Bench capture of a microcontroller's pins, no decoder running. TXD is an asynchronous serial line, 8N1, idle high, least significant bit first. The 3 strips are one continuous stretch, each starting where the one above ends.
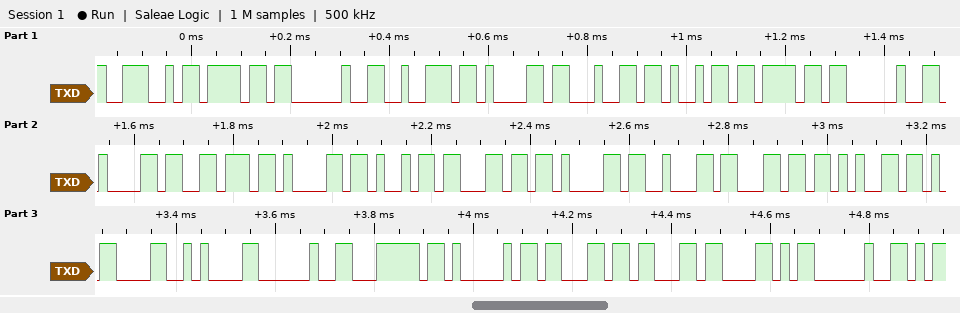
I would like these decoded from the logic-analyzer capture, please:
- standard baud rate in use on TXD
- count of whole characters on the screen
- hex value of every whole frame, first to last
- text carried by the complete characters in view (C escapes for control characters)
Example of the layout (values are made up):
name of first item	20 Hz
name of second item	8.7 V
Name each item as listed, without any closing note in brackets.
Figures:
standard baud rate in use on TXD	57600 baud
count of whole characters on the screen	27
hex value of every whole frame, first to last	0x4E 0x6F 0x20 0x72 0x61 0x64 0x69 0x6F 0x20 0x61 0x76 0x61 0x69 0x6C 0x61 0x62 0x6C 0x65 0x0D 0x0A 0x20 0x7C 0x41 0x63 0x63 0x58 0x20
text carried by the complete characters in view	"No radio available\r\n |AccX "
